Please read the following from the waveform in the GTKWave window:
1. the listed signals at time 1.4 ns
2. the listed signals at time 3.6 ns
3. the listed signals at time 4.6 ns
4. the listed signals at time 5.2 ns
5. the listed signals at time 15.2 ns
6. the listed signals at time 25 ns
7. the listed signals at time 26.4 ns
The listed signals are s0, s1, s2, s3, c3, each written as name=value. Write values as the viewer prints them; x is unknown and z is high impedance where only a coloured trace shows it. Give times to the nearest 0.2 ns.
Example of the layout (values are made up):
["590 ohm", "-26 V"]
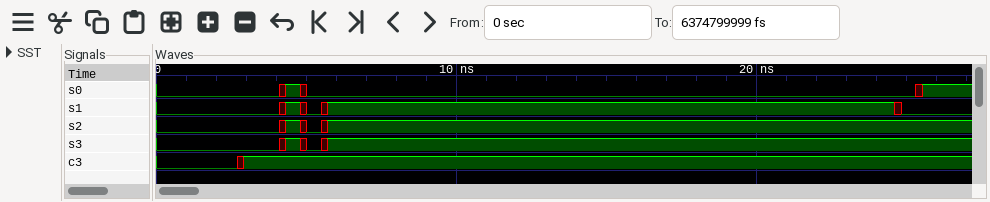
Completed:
["s0=0, s1=0, s2=0, s3=0, c3=0", "s0=0, s1=0, s2=0, s3=0, c3=1", "s0=1, s1=1, s2=1, s3=1, c3=1", "s0=0, s1=0, s2=0, s3=0, c3=1", "s0=0, s1=1, s2=1, s3=1, c3=1", "s0=0, s1=0, s2=1, s3=1, c3=1", "s0=1, s1=0, s2=1, s3=1, c3=1"]
